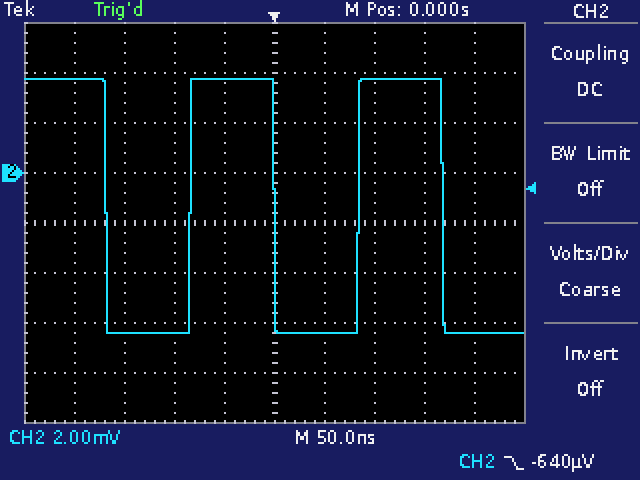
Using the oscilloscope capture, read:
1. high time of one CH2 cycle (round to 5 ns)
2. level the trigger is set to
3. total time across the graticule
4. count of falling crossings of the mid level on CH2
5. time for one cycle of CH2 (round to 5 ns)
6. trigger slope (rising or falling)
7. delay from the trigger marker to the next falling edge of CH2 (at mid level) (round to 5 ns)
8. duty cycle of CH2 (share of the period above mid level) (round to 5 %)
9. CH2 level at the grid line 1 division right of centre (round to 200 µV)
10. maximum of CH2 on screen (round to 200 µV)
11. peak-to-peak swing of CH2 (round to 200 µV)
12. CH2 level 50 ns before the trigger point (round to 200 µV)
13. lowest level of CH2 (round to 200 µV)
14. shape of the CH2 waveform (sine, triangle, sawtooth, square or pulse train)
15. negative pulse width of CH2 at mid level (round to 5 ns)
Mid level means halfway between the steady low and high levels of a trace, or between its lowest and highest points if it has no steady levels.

85 ns
-640 µV
500 ns
3
170 ns
falling
170 ns
50 %
-6.4 mV
3.8 mV
10.2 mV
3.8 mV
-6.4 mV
square
85 ns
